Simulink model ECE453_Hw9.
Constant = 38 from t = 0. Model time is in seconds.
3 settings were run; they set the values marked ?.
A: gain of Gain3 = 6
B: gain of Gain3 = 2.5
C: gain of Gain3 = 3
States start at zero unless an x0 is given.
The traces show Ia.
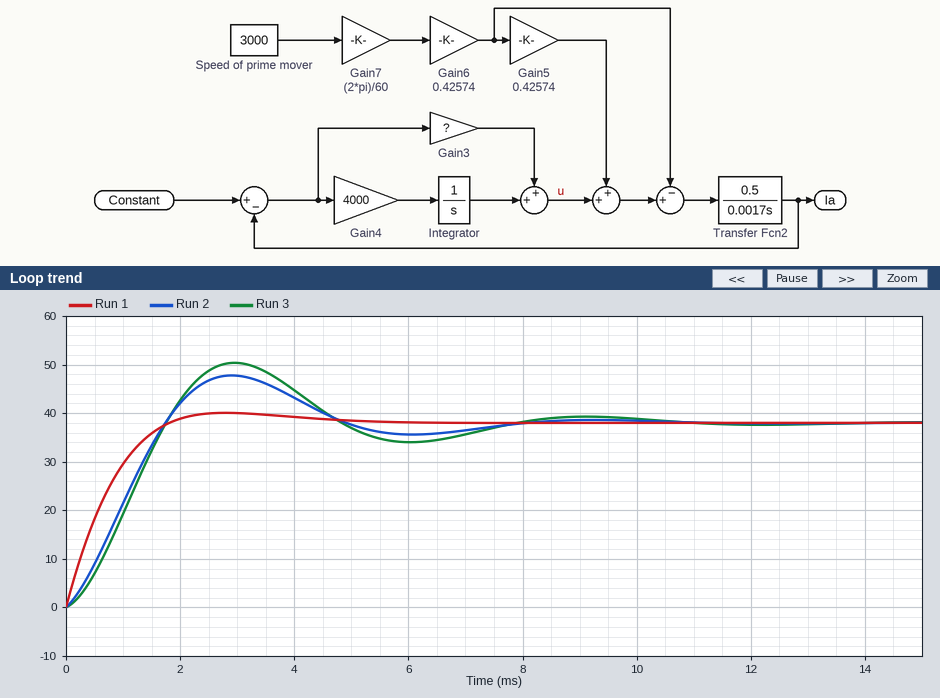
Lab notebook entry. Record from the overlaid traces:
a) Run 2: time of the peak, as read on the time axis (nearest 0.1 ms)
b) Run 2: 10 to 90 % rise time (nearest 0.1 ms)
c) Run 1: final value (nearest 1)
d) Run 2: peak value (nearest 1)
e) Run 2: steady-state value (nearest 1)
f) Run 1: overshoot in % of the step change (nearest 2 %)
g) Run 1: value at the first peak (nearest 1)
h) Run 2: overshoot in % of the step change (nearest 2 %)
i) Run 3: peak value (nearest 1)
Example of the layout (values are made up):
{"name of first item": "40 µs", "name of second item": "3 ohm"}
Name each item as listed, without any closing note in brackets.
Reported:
{"Run 2: time of the peak, as read on the time axis": "2.9 ms", "Run 2: 10 to 90 % rise time": "1.3 ms", "Run 1: final value": "38", "Run 2: peak value": "48", "Run 2: steady-state value": "38", "Run 1: overshoot in % of the step change": "6 %", "Run 1: value at the first peak": "40", "Run 2: overshoot in % of the step change": "26 %", "Run 3: peak value": "50"}
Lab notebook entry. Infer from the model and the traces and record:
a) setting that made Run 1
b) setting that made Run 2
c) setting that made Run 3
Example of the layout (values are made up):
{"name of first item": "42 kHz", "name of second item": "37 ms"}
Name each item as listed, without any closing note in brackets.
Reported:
{"setting that made Run 1": "A", "setting that made Run 2": "C", "setting that made Run 3": "B"}
